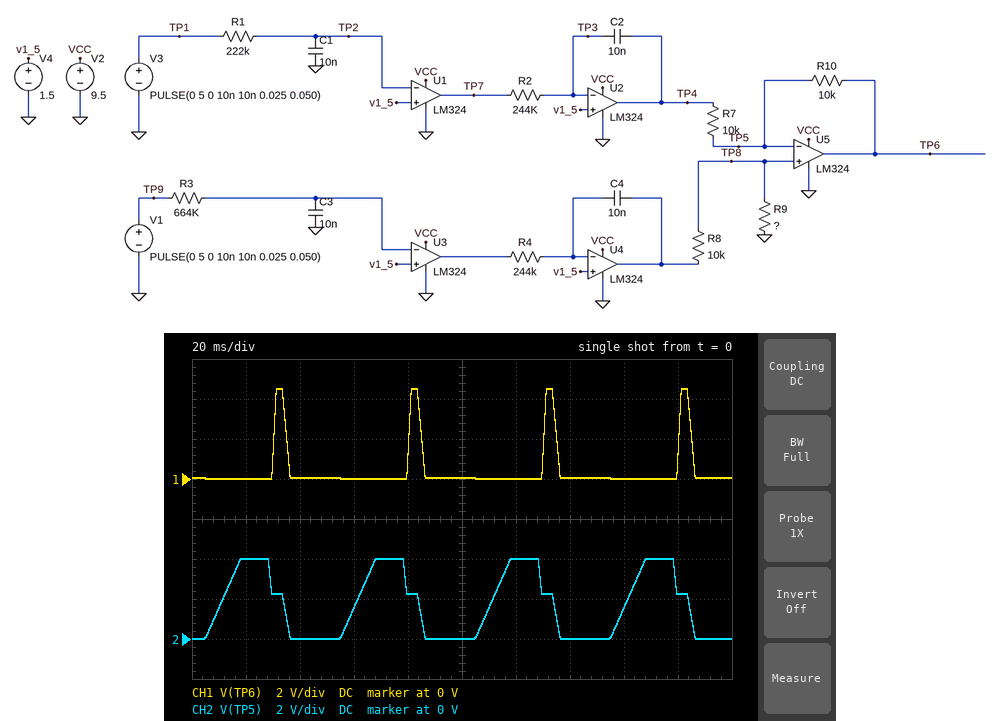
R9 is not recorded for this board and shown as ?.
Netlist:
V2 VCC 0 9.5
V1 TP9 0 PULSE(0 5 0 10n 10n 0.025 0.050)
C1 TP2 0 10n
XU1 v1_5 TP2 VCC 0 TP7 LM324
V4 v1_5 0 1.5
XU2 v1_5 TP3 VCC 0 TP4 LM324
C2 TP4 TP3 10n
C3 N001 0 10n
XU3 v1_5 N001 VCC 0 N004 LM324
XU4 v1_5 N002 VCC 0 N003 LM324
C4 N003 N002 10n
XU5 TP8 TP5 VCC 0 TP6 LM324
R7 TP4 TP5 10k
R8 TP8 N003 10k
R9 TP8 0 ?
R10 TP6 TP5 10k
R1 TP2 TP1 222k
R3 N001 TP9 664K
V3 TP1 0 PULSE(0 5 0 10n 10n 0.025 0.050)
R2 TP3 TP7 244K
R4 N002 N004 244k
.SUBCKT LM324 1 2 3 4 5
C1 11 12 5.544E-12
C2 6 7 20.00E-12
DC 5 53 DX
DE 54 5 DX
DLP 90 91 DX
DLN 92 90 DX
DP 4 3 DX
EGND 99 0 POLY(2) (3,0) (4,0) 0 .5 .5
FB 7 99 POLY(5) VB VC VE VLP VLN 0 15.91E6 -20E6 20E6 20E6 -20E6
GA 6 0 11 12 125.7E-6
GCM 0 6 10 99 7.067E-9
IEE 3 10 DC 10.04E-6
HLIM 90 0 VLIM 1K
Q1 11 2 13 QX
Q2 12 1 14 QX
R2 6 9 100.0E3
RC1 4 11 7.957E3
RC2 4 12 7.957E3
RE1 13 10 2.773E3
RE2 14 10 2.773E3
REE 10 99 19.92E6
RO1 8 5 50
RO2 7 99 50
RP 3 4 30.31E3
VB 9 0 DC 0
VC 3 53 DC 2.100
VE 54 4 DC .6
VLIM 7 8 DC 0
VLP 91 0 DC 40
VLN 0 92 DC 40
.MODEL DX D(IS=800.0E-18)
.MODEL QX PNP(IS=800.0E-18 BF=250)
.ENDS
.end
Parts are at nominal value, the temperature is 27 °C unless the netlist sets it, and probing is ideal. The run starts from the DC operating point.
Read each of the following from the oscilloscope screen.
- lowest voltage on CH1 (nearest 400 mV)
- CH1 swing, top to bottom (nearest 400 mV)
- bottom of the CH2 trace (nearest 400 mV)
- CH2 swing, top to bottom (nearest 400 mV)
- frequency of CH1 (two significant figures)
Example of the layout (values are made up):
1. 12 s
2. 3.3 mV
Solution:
1. 0 V
2. 4.4 V
3. 0 V
4. 4.0 V
5. 20 Hz
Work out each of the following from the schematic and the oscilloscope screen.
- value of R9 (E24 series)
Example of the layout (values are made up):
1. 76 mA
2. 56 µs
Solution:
1. 3.9 kΩ
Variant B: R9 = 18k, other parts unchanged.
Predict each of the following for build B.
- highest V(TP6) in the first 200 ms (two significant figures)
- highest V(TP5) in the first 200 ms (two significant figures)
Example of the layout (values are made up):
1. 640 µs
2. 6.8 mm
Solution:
1. 8.0 V
2. 5.1 V
